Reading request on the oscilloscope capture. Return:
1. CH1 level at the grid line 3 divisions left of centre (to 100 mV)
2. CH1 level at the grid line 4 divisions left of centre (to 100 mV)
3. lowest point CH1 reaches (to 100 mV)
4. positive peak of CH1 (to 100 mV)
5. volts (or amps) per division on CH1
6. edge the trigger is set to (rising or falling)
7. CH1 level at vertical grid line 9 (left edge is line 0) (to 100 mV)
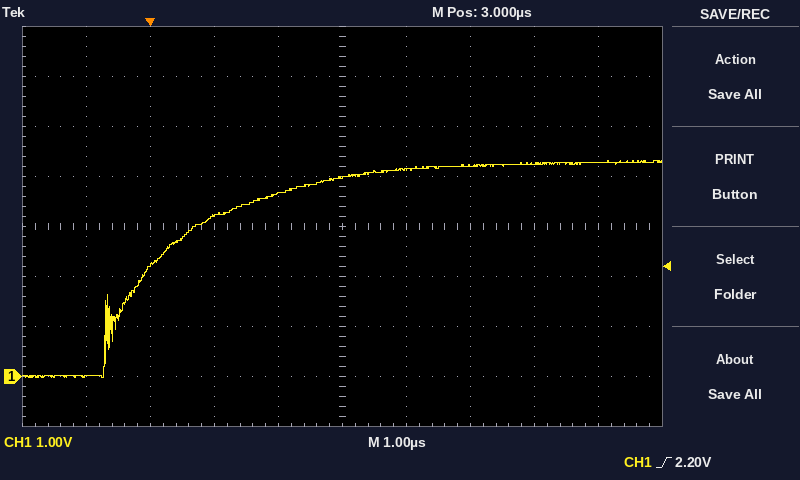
2.2 V
0.0 V
0.0 V
4.3 V
1 V
rising
4.3 V
